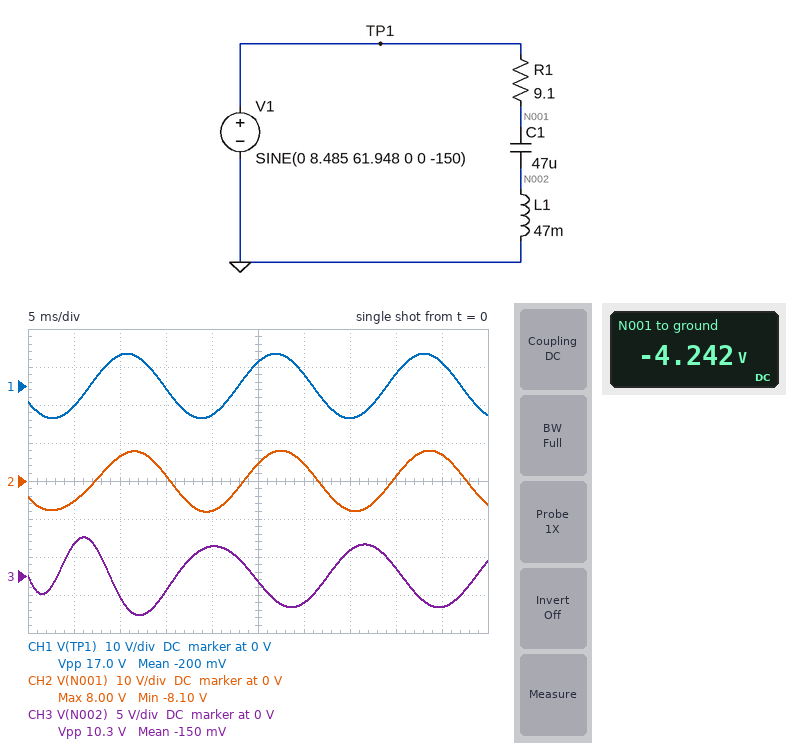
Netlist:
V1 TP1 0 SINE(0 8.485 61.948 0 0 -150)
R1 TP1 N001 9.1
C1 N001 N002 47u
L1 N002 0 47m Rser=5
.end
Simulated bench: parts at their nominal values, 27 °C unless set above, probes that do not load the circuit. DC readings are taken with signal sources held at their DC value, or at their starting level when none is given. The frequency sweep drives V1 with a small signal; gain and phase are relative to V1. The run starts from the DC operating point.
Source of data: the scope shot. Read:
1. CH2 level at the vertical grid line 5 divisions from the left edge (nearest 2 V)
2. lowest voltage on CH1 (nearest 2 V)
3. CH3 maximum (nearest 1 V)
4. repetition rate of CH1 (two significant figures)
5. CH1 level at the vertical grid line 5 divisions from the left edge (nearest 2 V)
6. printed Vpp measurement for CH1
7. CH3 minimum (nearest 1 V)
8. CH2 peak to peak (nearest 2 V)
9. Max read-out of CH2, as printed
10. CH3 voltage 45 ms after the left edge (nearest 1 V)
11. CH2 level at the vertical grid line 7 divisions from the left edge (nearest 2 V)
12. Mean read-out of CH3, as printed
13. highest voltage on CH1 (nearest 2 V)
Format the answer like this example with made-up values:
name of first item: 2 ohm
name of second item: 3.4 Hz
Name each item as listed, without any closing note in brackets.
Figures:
CH2 level at the vertical grid line 5 divisions from the left edge: 4 V
lowest voltage on CH1: -8 V
CH3 maximum: 5 V
repetition rate of CH1: 62 Hz
CH1 level at the vertical grid line 5 divisions from the left edge: 6 V
printed Vpp measurement for CH1: 17.0 V
CH3 minimum: -5 V
CH2 peak to peak: 16 V
Max read-out of CH2, as printed: 8.00 V
CH3 voltage 45 ms after the left edge: -4 V
CH2 level at the vertical grid line 7 divisions from the left edge: -8 V
Mean read-out of CH3, as printed: -150 mV
highest voltage on CH1: 8 V
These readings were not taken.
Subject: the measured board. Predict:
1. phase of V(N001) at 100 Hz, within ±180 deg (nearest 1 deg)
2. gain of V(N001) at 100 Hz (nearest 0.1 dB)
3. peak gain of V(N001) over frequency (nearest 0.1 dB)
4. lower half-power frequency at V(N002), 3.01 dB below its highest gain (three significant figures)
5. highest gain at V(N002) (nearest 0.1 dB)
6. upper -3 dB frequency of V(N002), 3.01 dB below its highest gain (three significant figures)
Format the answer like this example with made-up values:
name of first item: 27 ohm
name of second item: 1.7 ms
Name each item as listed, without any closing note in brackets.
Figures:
phase of V(N001) at 100 Hz, within ±180 deg: -24 deg
gain of V(N001) at 100 Hz: -7.0 dB
peak gain of V(N001) over frequency: 0 dB
lower half-power frequency at V(N002), 3.01 dB below its highest gain: 92.5 Hz
highest gain at V(N002): 7.3 dB
upper -3 dB frequency of V(N002), 3.01 dB below its highest gain: 156 Hz
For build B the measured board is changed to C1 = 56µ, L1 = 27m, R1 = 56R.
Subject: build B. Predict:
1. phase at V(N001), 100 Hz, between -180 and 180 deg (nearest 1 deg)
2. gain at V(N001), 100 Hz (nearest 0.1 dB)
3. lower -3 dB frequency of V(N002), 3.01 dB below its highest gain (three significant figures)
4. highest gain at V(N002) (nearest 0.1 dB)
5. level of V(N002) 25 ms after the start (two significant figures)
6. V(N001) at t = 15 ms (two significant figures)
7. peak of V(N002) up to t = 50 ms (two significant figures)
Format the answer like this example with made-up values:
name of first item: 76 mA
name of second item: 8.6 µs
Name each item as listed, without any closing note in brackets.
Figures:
phase at V(N001), 100 Hz, between -180 and 180 deg: -56 deg
gain at V(N001), 100 Hz: -13.9 dB
lower -3 dB frequency of V(N002), 3.01 dB below its highest gain: 311 Hz
highest gain at V(N002): 0 dB
level of V(N002) 25 ms after the start: 860 mV
V(N001) at t = 15 ms: 3.1 V
peak of V(N002) up to t = 50 ms: 1.4 V
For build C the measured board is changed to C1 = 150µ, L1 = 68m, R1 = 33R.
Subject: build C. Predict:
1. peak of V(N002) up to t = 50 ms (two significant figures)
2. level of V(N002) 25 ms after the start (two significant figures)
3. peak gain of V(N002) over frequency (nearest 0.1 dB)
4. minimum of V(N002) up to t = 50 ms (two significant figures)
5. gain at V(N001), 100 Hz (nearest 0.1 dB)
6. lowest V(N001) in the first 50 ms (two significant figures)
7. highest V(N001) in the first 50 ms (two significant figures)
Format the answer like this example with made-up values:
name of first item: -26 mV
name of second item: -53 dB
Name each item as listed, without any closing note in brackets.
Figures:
peak of V(N002) up to t = 50 ms: 5.8 V
level of V(N002) 25 ms after the start: 5.4 V
peak gain of V(N002) over frequency: 0 dB
minimum of V(N002) up to t = 50 ms: -6.0 V
gain at V(N001), 100 Hz: -3.7 dB
lowest V(N001) in the first 50 ms: -6.7 V
highest V(N001) in the first 50 ms: 2.3 V
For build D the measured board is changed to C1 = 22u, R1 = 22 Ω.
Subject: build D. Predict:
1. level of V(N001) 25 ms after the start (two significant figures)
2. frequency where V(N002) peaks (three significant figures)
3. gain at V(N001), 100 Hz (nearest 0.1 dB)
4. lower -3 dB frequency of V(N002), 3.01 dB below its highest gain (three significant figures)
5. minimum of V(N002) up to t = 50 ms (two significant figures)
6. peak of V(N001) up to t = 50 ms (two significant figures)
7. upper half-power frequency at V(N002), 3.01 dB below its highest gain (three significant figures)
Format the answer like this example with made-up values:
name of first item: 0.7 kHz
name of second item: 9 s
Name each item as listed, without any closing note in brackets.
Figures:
level of V(N001) 25 ms after the start: 4.7 V
frequency where V(N002) peaks: 172 Hz
gain at V(N001), 100 Hz: -1.4 dB
lower -3 dB frequency of V(N002), 3.01 dB below its highest gain: 133 Hz
minimum of V(N002) up to t = 50 ms: -1.7 V
peak of V(N001) up to t = 50 ms: 8.2 V
upper half-power frequency at V(N002), 3.01 dB below its highest gain: 299 Hz
